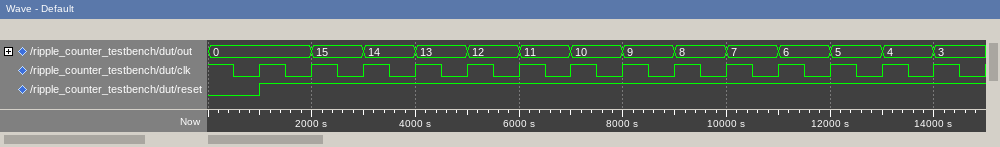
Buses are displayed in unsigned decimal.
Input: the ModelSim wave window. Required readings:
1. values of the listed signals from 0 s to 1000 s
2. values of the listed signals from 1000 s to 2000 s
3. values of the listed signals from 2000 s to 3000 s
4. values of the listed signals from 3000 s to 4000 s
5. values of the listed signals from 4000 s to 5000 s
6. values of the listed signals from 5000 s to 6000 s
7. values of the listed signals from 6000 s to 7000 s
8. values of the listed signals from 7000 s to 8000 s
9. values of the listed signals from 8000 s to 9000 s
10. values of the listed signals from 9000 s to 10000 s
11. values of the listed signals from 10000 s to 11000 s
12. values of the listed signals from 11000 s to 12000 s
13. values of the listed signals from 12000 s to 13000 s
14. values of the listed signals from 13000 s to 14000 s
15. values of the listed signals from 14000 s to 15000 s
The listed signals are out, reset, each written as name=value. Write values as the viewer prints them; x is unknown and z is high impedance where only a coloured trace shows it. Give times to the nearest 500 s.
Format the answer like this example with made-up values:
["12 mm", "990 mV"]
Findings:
["out=0, reset=0", "out=0, reset=1", "out=15, reset=1", "out=14, reset=1", "out=13, reset=1", "out=12, reset=1", "out=11, reset=1", "out=10, reset=1", "out=9, reset=1", "out=8, reset=1", "out=7, reset=1", "out=6, reset=1", "out=5, reset=1", "out=4, reset=1", "out=3, reset=1"]
